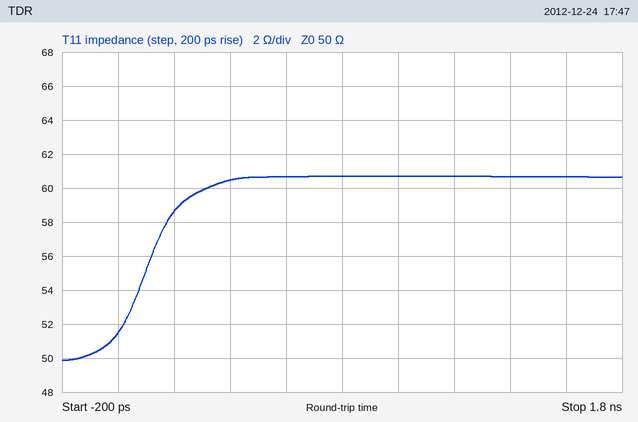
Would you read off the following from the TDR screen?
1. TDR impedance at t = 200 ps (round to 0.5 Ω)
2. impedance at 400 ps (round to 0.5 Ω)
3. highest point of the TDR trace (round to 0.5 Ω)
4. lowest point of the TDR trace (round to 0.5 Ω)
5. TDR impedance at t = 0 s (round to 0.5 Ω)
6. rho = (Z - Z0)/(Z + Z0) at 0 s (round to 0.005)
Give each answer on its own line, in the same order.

58.5 Ω
60.5 Ω
60.5 Ω
50.0 Ω
51.5 Ω
+0.015
